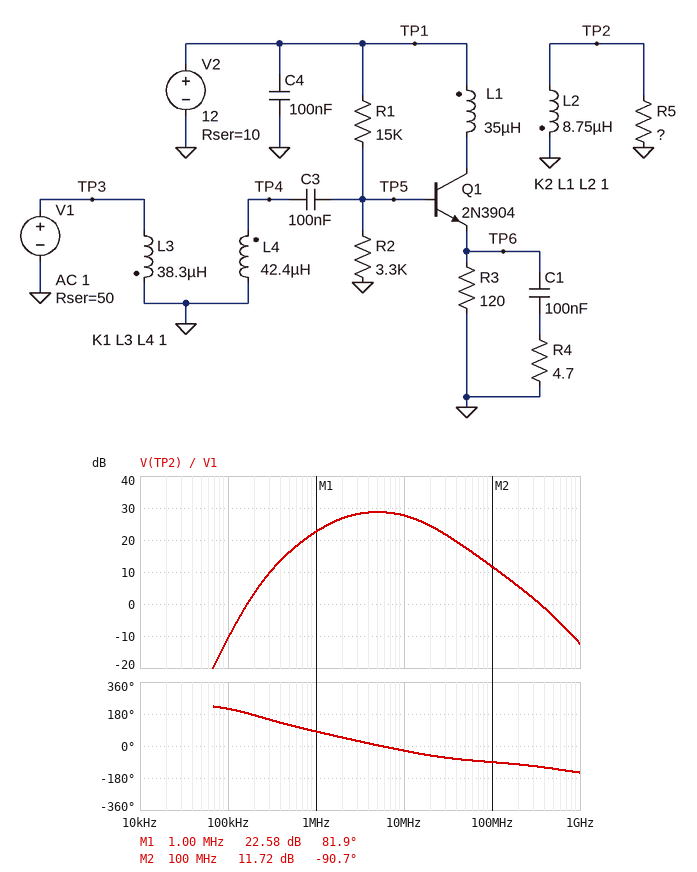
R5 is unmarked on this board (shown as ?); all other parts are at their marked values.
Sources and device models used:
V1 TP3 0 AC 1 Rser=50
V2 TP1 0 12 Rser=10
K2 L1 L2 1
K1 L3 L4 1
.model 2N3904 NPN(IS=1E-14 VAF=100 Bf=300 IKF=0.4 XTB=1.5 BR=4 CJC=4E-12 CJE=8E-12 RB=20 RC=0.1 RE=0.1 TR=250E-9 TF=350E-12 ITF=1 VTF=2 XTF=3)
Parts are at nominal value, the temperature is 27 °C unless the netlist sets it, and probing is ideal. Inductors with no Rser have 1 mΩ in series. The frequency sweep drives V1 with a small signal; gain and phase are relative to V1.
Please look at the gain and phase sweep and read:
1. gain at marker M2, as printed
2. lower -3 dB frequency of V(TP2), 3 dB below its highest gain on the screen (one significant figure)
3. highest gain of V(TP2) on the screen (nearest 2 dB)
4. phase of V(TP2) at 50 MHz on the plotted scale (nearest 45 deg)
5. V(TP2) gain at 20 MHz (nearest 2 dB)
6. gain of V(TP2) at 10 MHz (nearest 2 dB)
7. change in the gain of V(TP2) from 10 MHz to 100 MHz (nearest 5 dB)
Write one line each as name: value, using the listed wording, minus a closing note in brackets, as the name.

gain at marker M2, as printed: 11.72 dB
lower -3 dB frequency of V(TP2), 3 dB below its highest gain on the screen: 2 MHz
highest gain of V(TP2) on the screen: 28 dB
phase of V(TP2) at 50 MHz on the plotted scale: -90 deg
V(TP2) gain at 20 MHz: 24 dB
gain of V(TP2) at 10 MHz: 28 dB
change in the gain of V(TP2) from 10 MHz to 100 MHz: -15 dB
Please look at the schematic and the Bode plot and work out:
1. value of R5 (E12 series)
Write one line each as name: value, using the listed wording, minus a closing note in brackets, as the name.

value of R5: 100 Ω
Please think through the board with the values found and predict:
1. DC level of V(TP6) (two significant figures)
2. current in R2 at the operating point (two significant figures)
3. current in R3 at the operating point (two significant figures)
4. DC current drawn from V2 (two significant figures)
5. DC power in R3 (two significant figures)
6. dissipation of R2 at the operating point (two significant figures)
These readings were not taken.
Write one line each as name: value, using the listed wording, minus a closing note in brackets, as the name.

DC level of V(TP6): 1.3 V
current in R2 at the operating point: 620 µA
current in R3 at the operating point: 11 mA
DC current drawn from V2: 12 mA
DC power in R3: 15 mW
dissipation of R2 at the operating point: 1.3 mW
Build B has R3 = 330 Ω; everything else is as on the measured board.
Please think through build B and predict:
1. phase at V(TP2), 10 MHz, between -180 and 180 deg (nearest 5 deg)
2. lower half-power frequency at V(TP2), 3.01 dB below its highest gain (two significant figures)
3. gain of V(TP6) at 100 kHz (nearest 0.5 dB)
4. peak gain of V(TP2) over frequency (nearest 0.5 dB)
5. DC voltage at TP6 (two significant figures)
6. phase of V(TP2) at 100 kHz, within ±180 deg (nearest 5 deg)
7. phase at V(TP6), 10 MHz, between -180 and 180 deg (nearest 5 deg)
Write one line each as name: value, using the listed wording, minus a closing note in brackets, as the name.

phase at V(TP2), 10 MHz, between -180 and 180 deg: -15 deg
lower half-power frequency at V(TP2), 3.01 dB below its highest gain: 1.7 MHz
gain of V(TP6) at 100 kHz: -8.5 dB
peak gain of V(TP2) over frequency: 25.0 dB
DC voltage at TP6: 1.4 V
phase of V(TP2) at 100 kHz, within ±180 deg: -155 deg
phase at V(TP6), 10 MHz, between -180 and 180 deg: 155 deg
